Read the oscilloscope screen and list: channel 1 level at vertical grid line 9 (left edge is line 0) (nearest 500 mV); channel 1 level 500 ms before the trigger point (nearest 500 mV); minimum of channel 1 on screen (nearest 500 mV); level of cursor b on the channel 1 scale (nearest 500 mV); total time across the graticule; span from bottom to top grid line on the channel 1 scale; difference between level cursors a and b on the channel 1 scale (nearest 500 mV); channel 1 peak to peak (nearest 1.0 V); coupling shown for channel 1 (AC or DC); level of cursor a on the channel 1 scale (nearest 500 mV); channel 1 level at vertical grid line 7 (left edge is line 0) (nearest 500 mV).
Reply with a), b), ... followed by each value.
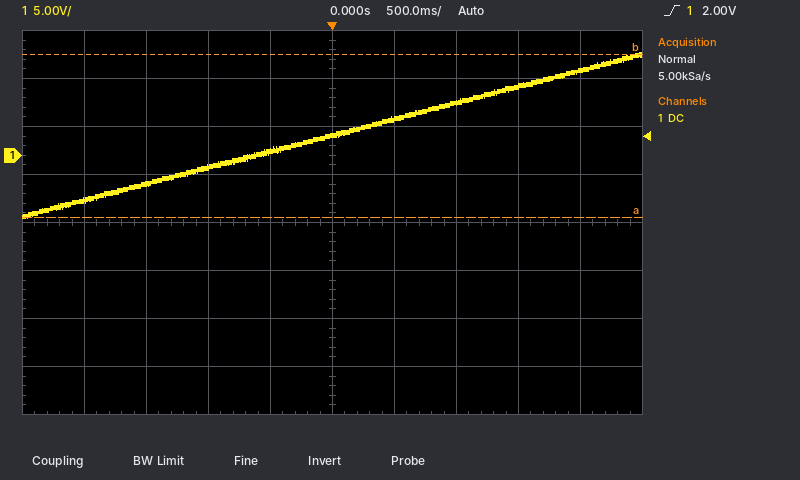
a) 9.0 V
b) 500 mV
c) -6.5 V
d) 10.5 V
e) 5 s
f) 40 V
g) 17.0 V
h) 17.0 V
i) DC
j) -6.5 V
k) 5.5 V
